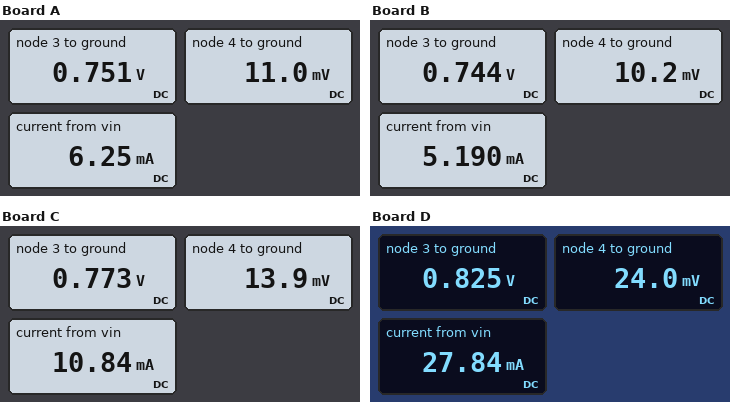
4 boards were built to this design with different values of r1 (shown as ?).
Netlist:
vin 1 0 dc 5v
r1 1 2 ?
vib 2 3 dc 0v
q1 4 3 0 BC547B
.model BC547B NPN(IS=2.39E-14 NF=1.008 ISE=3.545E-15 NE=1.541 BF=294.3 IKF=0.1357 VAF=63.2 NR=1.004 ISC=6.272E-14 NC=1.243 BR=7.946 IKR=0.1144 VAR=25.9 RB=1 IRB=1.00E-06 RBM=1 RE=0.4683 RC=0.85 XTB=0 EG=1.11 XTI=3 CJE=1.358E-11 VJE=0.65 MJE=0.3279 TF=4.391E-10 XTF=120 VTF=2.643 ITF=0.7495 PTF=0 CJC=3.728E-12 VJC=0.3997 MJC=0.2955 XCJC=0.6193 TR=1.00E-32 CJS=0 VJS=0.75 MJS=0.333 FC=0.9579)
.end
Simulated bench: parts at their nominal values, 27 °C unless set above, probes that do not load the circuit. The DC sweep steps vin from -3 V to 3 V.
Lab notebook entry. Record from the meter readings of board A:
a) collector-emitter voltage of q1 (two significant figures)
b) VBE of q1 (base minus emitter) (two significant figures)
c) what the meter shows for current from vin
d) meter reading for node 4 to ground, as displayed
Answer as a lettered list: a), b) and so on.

a) 11 mV
b) 750 mV
c) 6.25 mA
d) 11.0 mV
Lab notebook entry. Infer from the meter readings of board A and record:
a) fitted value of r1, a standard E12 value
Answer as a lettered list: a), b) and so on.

a) 680 Ω
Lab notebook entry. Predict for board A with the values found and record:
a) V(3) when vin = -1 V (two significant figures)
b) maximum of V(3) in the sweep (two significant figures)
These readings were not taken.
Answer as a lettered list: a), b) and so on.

a) -1.0 V
b) 730 mV
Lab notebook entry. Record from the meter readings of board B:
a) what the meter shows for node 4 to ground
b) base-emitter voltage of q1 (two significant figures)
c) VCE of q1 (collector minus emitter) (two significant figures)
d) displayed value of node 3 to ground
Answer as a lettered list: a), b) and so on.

a) 10.2 mV
b) 740 mV
c) 10 mV
d) 0.744 V
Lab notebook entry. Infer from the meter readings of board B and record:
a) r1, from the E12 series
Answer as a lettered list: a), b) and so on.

a) 820 Ω
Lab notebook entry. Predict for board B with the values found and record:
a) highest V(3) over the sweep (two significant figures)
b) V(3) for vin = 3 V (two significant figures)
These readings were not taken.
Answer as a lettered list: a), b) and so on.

a) 720 mV
b) 720 mV
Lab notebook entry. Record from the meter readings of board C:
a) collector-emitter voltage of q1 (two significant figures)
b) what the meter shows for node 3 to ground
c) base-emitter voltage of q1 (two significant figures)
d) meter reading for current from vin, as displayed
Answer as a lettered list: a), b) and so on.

a) 14 mV
b) 0.773 V
c) 770 mV
d) 10.84 mA
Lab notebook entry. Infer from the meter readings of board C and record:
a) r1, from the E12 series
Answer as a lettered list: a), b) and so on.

a) 390 Ω
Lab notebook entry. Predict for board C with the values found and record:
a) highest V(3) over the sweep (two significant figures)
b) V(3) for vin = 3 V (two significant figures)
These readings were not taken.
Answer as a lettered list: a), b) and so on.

a) 750 mV
b) 750 mV
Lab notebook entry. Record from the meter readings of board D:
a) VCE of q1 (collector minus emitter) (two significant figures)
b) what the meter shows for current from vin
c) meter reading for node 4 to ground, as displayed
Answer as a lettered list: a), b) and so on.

a) 24 mV
b) 27.84 mA
c) 24.0 mV
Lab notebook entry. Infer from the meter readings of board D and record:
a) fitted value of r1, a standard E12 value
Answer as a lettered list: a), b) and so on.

a) 150 Ω
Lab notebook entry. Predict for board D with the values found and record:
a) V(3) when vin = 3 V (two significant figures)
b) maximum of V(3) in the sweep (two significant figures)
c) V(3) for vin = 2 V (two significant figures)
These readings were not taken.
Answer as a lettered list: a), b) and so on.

a) 790 mV
b) 790 mV
c) 760 mV
